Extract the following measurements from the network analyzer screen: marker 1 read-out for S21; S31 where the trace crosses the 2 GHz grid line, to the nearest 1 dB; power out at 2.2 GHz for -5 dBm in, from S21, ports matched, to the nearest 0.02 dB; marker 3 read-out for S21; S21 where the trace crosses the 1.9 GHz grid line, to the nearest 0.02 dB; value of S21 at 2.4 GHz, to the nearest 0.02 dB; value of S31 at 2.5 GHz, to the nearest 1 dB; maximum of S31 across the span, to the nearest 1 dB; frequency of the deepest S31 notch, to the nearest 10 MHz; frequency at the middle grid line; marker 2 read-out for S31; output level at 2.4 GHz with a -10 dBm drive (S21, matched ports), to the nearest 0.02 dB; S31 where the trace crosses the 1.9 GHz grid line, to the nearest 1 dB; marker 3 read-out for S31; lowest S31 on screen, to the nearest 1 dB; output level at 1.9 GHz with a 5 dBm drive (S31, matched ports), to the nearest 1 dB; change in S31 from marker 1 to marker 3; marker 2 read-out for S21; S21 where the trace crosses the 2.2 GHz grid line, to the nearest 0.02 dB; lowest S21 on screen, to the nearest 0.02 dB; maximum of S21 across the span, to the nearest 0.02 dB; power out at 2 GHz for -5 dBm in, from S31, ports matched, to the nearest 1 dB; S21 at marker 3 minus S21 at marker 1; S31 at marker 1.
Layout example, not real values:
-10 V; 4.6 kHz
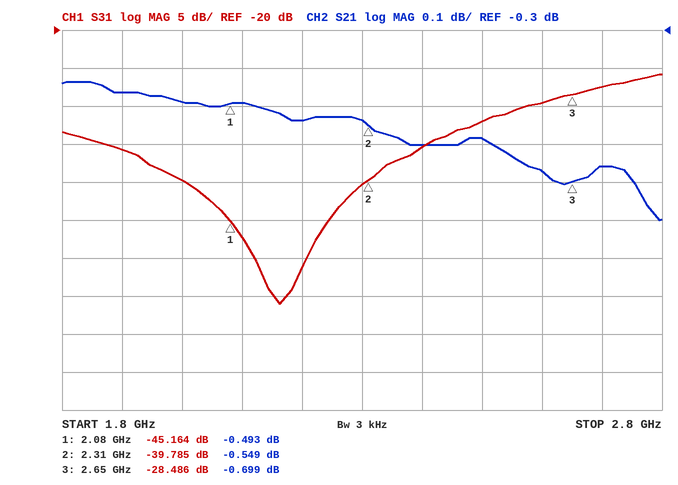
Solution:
-0.493 dB; -40 dB; -5.54 dBm; -0.699 dB; -0.46 dB; -0.60 dB; -32 dB; -26 dB; 2.16 GHz; 2.3 GHz; -39.785 dB; -10.60 dBm; -36 dB; -28.486 dB; -56 dB; -31 dBm; 16.678 dB; -0.549 dB; -0.54 dB; -0.80 dB; -0.44 dB; -45 dBm; -0.206 dB; -45.164 dB
